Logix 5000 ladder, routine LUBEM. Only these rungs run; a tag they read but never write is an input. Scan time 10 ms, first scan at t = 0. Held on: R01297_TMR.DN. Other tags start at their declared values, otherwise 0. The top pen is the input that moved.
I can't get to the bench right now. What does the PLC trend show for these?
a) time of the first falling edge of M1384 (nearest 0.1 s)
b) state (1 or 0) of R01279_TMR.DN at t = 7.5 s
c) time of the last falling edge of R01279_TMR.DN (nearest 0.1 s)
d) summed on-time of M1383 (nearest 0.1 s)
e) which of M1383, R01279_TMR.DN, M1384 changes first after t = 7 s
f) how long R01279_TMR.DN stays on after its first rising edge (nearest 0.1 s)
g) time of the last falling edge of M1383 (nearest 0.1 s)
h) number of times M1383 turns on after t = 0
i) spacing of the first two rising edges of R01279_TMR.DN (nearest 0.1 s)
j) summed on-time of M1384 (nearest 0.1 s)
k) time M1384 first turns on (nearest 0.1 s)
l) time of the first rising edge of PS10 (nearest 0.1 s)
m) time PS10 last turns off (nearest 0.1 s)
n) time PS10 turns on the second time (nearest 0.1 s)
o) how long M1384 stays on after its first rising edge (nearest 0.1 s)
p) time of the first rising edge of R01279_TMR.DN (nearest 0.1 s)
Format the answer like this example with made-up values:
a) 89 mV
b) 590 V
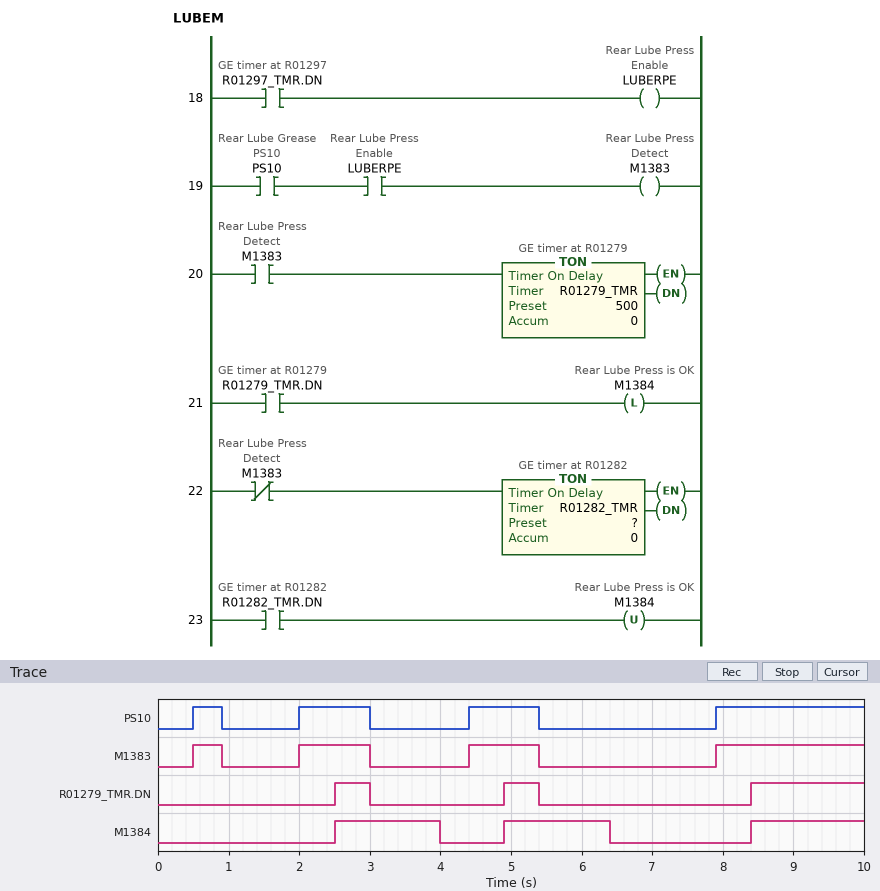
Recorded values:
a) 4.0 s
b) 0
c) 5.4 s
d) 4.5 s
e) M1383
f) 0.5 s
g) 5.4 s
h) 4
i) 2.4 s
j) 4.6 s
k) 2.5 s
l) 0.5 s
m) 5.4 s
n) 2.0 s
o) 1.5 s
p) 2.5 s
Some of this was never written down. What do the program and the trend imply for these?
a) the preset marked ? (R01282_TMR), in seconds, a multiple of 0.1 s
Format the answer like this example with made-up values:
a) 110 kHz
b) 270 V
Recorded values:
a) 1.0 s
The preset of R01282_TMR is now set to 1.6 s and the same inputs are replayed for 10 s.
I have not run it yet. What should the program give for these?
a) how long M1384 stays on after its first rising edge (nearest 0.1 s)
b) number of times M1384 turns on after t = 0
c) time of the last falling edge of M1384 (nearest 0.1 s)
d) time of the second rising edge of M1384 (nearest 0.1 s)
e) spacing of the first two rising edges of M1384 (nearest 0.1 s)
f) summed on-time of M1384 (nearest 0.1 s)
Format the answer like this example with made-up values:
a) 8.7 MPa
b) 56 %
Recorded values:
a) 4.5 s
b) 2
c) 7.0 s
d) 8.4 s
e) 5.9 s
f) 6.1 s
